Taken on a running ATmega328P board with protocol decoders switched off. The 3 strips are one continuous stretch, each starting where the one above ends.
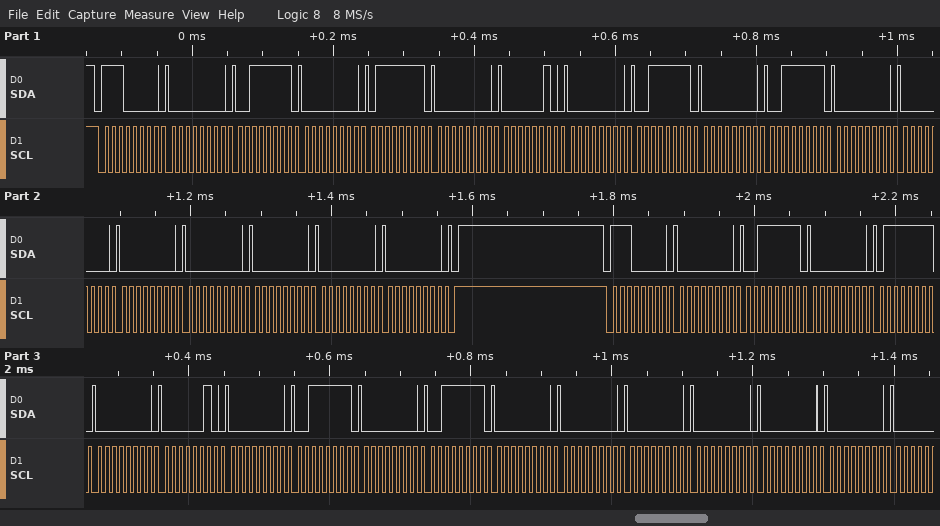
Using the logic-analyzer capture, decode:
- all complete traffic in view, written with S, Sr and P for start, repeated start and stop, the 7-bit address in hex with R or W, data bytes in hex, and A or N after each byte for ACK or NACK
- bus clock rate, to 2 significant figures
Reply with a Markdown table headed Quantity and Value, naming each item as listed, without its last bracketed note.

| Quantity | Value |
|---|---|
| all complete traffic in view, written with S, Sr and P for start, repeated start and stop, the 7-bit address in hex with R or W, data bytes in hex, and A or N after each byte for ACK or NACK | S 70W A 00 A 3F A 00 A 7F A 00 A 02 A 00 A 3F A 00 A 3F A 00 A 00 A 00 A 00 A 00 A 00 A 00 A P S 70W A 00 A 3F A 00 A 7F A 00 A 02 A 00 A 3F A 00 A 3F A 00 A 00 A 00 A 00 A 00 A 00 A |
| bus clock rate, to 2 significant figures | 100 kHz |
